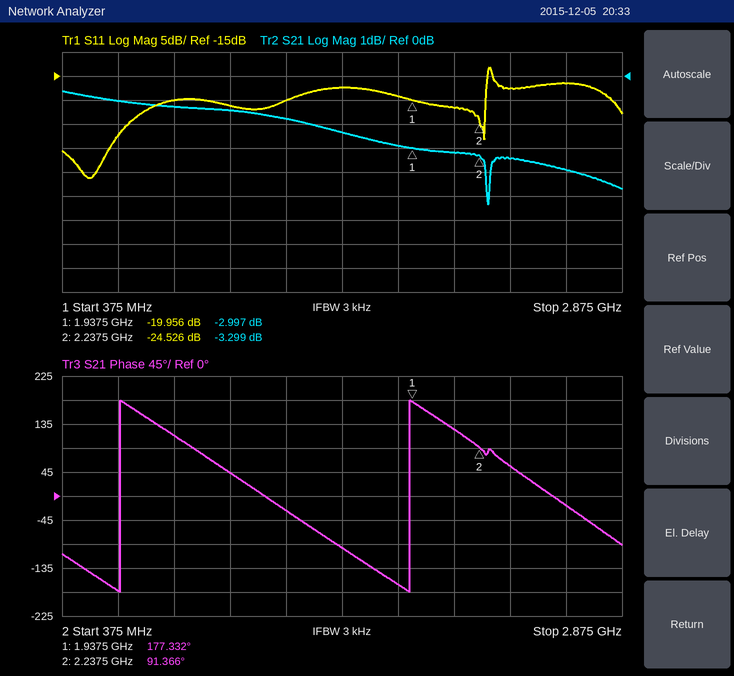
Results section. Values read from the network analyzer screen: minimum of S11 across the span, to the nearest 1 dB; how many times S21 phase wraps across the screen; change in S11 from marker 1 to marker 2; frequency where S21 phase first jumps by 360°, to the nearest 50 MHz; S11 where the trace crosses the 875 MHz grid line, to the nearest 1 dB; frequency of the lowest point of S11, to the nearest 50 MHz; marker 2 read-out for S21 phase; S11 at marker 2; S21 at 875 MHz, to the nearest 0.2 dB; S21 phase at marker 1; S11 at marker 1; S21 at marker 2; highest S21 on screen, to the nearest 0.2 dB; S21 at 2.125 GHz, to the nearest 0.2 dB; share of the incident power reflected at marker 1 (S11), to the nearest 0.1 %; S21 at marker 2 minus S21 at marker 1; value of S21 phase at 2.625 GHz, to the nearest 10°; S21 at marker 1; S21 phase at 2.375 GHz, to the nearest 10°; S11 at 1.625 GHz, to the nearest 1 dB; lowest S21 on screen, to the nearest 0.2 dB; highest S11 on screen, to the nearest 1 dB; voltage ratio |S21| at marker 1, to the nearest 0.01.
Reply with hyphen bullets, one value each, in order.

- -36 dB
- 2
- -4.570 dB
- 650 MHz
- -20 dB
- 500 MHz
- 91.366°
- -24.526 dB
- -1.2 dB
- 177.332°
- -19.956 dB
- -3.299 dB
- -0.6 dB
- -3.2 dB
- 1.0 %
- -0.302 dB
- -20°
- -2.997 dB
- 60°
- -17 dB
- -5.4 dB
- -13 dB
- 0.71
